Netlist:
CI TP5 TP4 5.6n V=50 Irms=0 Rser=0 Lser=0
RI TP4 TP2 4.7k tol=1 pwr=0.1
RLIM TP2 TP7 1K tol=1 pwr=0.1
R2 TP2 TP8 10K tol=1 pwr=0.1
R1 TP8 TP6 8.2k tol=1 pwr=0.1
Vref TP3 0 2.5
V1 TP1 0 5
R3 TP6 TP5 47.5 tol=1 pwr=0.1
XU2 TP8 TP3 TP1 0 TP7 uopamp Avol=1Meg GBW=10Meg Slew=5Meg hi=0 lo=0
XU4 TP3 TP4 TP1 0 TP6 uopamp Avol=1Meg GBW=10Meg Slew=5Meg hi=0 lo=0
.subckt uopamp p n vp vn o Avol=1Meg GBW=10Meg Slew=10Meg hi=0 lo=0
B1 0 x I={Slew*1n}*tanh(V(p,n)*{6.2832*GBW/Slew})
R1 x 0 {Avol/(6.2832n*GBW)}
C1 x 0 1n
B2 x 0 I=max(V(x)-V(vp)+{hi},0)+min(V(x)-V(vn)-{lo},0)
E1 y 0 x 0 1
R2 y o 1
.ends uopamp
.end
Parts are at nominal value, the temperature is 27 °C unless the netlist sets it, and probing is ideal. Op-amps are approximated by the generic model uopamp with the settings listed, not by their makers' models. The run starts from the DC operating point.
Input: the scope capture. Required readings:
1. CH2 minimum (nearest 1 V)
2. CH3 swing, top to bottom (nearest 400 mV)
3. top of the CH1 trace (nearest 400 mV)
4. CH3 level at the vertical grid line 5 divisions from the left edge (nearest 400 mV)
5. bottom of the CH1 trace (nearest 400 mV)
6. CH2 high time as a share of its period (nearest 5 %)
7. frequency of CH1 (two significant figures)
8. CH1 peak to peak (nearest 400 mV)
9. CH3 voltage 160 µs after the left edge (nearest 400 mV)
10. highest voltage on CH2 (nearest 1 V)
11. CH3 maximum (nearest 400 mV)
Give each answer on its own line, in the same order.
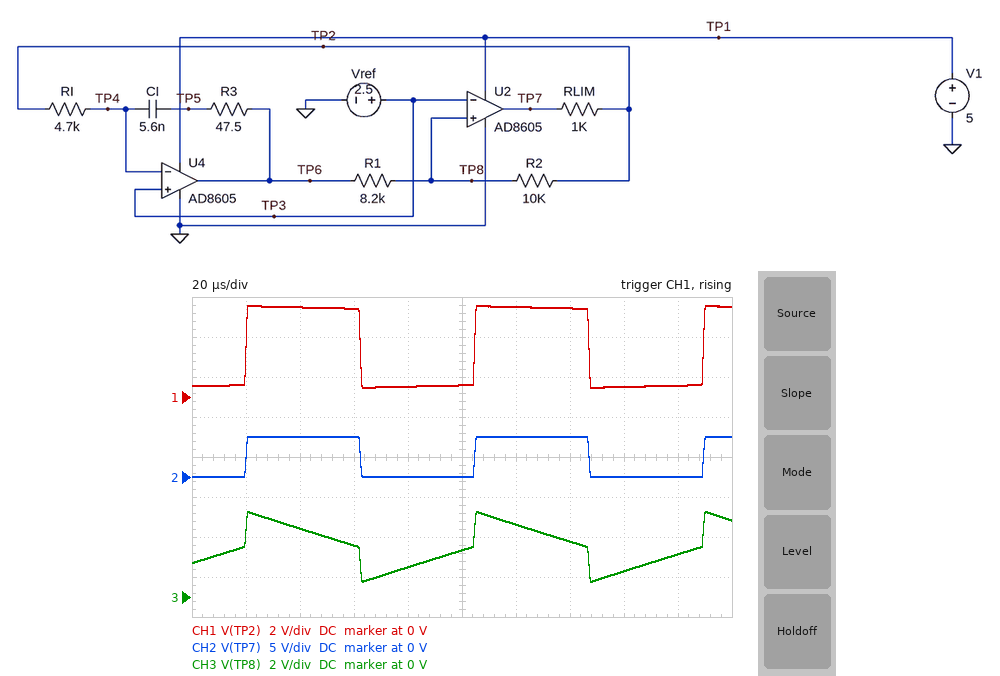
0 V
3.6 V
4.4 V
2.4 V
400 mV
50 %
12 kHz
4.0 V
1.2 V
5 V
4.4 V
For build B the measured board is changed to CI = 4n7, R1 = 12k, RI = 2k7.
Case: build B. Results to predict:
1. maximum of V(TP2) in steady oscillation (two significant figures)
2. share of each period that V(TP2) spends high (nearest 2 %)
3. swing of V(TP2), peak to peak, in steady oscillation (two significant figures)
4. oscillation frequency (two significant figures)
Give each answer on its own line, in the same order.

4.3 V
50 %
3.7 V
17 kHz
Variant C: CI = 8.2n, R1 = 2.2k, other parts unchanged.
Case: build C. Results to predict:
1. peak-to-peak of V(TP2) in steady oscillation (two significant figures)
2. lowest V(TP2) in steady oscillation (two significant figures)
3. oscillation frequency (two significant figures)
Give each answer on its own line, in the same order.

3.9 V
540 mV
29 kHz
